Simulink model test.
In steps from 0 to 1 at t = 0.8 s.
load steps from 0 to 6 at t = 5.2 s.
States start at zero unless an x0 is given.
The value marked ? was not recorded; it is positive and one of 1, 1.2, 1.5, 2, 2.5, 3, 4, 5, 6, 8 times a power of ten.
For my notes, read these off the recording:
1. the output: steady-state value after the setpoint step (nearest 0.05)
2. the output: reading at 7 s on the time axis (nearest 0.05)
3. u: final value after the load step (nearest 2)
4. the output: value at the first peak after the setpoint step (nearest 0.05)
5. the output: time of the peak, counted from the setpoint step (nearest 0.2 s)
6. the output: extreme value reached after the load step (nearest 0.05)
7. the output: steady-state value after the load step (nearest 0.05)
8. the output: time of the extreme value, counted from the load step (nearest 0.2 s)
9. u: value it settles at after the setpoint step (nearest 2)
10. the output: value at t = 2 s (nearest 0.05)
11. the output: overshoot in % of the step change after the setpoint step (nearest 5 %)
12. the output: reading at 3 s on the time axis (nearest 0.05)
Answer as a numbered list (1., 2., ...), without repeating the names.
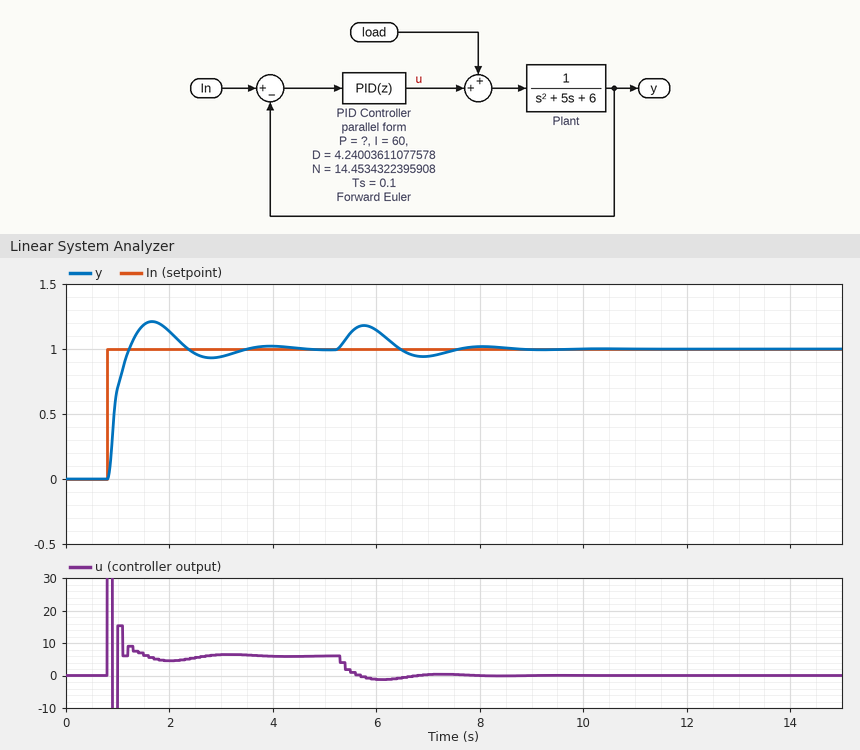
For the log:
1. 1.00
2. 0.95
3. 0
4. 1.20
5. 0.8 s
6. 1.20
7. 1.00
8. 0.6 s
9. 6
10. 1.15
11. 20 %
12. 0.95
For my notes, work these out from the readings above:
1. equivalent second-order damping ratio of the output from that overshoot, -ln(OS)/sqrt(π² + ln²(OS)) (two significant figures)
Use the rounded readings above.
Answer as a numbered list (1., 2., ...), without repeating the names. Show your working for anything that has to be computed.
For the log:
1. ln(0.2) = -1.609; 1.609 / sqrt(9.870 + 2.590) = 0.46
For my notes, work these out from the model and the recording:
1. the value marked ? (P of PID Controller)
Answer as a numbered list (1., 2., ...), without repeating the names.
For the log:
1. 20
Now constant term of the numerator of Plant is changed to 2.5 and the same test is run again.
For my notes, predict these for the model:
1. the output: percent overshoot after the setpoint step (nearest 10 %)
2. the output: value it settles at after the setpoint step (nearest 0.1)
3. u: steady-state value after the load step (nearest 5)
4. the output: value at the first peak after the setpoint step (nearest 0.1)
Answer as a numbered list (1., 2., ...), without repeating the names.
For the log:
1. 40 %
2. 1.0
3. -5
4. 1.4
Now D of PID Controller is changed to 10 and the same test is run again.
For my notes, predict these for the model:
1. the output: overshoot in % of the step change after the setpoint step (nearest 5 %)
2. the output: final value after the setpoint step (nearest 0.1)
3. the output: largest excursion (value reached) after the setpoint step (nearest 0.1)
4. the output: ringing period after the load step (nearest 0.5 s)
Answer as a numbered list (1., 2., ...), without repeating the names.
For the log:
1. 10 %
2. 1.0
3. 1.1
4. 3.0 s
